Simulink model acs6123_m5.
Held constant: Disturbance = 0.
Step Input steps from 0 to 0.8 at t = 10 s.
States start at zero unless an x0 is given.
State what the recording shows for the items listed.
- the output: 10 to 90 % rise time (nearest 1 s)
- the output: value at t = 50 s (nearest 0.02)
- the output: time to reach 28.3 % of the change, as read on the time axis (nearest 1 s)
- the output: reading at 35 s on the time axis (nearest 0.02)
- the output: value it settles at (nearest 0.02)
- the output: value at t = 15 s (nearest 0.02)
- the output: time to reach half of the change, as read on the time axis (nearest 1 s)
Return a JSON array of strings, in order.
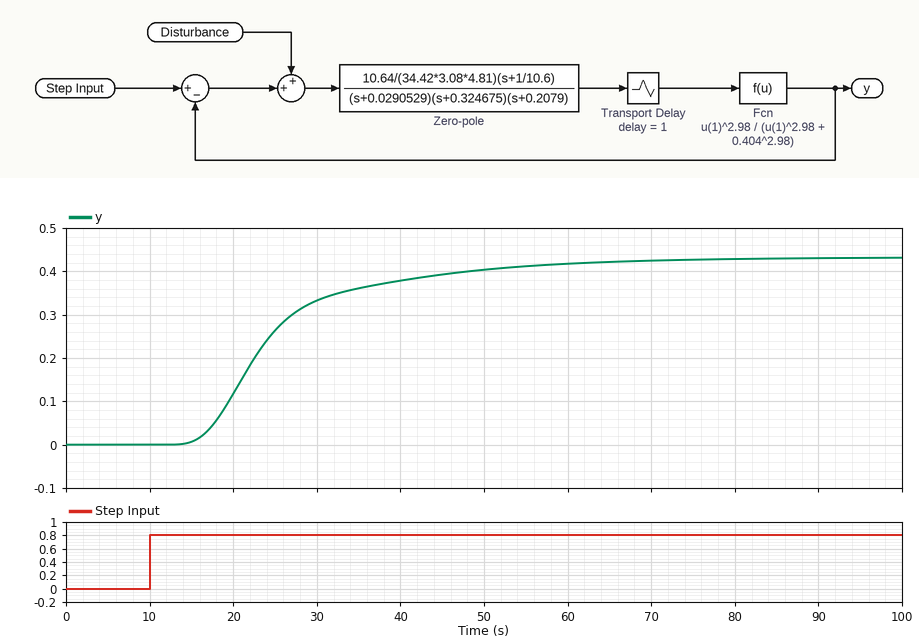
["26 s", "0.40", "20 s", "0.36", "0.44", "0.00", "23 s"]
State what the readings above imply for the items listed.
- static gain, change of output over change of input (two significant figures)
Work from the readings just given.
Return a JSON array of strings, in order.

["0.55"]
